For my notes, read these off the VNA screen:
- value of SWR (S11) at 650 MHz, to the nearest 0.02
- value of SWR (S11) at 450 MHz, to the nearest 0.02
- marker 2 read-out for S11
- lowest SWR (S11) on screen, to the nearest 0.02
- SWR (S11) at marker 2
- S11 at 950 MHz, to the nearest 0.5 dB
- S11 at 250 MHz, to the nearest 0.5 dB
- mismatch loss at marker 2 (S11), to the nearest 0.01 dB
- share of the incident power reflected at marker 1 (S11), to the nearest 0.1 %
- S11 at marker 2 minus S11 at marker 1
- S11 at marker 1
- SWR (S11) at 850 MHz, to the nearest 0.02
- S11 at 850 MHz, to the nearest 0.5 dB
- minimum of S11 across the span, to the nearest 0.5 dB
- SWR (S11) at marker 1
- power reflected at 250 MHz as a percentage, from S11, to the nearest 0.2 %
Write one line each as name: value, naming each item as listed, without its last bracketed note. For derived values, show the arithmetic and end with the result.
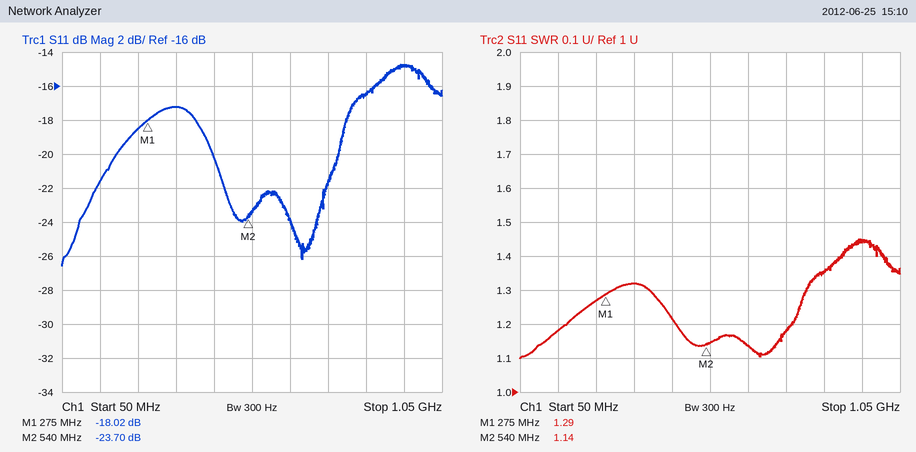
value of SWR (S11) at 650 MHz, to the nearest 0.02: 1.14
value of SWR (S11) at 450 MHz, to the nearest 0.02: 1.22
marker 2 read-out for S11: -23.70 dB
lowest SWR (S11) on screen, to the nearest 0.02: 1.10
SWR (S11) at marker 2: 1.14
S11 at 950 MHz, to the nearest 0.5 dB: -15.0 dB
S11 at 250 MHz, to the nearest 0.5 dB: -18.5 dB
mismatch loss at marker 2 (S11), to the nearest 0.01 dB: −10 log10(1 − 10^(-23.7/10)) ≈ 0.02 dB
share of the incident power reflected at marker 1 (S11), to the nearest 0.1 %: 10^(-18.02/10) ≈ 1.6 %
S11 at marker 2 minus S11 at marker 1: -23.7 − (-18.02) = -5.68 dB
S11 at marker 1: -18.02 dB
SWR (S11) at 850 MHz, to the nearest 0.02: 1.36
S11 at 850 MHz, to the nearest 0.5 dB: -16.5 dB
minimum of S11 across the span, to the nearest 0.5 dB: -26.5 dB
SWR (S11) at marker 1: 1.29
power reflected at 250 MHz as a percentage, from S11, to the nearest 0.2 %: 10^(-18.5/10) ≈ 1.4 %
